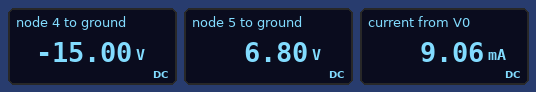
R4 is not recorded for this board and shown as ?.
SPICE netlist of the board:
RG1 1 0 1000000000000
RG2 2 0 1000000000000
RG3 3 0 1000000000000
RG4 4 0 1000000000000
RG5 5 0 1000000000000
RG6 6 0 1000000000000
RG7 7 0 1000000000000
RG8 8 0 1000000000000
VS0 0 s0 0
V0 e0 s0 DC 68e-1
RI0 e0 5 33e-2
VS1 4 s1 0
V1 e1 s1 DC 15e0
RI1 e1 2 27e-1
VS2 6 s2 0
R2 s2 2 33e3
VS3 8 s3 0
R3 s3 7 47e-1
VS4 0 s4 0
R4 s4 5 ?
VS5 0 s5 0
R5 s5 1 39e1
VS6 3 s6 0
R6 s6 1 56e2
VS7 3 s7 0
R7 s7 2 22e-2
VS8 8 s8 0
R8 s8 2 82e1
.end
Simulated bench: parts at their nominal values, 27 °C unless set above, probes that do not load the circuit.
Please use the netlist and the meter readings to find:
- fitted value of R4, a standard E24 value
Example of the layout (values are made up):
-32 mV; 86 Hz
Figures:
750 Ω
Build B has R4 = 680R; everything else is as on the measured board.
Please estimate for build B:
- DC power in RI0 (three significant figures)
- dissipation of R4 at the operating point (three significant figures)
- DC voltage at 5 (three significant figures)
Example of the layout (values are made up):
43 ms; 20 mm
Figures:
33.0 µW; 67.9 mW; 6.80 V
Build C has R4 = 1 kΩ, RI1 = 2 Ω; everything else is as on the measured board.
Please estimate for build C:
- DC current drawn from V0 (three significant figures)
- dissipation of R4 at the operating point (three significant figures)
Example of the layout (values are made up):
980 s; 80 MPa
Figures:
6.80 mA; 46.2 mW
